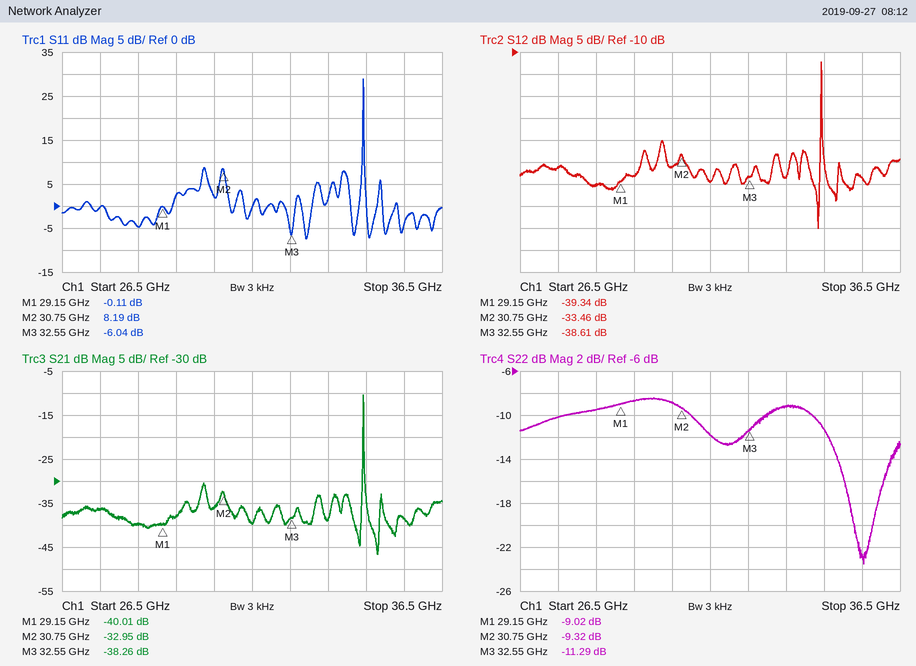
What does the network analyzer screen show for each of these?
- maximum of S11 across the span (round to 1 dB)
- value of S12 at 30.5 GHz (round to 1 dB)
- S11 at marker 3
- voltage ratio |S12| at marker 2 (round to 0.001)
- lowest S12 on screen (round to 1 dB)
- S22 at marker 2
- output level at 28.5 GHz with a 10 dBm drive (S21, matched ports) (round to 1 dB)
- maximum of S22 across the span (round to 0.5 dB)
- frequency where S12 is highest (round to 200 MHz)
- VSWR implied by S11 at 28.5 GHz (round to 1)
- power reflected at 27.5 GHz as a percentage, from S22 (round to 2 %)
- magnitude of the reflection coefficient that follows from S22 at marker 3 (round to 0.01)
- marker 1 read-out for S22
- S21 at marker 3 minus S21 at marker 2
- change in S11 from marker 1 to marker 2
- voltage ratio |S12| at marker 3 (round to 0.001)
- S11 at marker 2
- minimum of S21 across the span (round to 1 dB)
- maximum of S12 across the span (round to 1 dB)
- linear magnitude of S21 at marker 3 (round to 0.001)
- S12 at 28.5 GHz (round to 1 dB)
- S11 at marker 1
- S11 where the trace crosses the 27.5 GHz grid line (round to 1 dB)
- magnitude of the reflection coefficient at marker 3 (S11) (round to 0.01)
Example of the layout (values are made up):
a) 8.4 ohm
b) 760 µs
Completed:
a) 29 dB
b) -36 dB
c) -6.04 dB
d) 0.021
e) -50 dB
f) -9.32 dB
g) -30 dBm
h) -8.5 dB
i) 34.4 GHz
j) 4
k) 10 %
l) 0.27
m) -9.02 dB
n) -5.31 dB
o) 8.30 dB
p) 0.012
q) 8.19 dB
r) -47 dB
s) -12 dB
t) 0.012
u) -40 dB
v) -0.11 dB
w) 0 dB
x) 0.50
